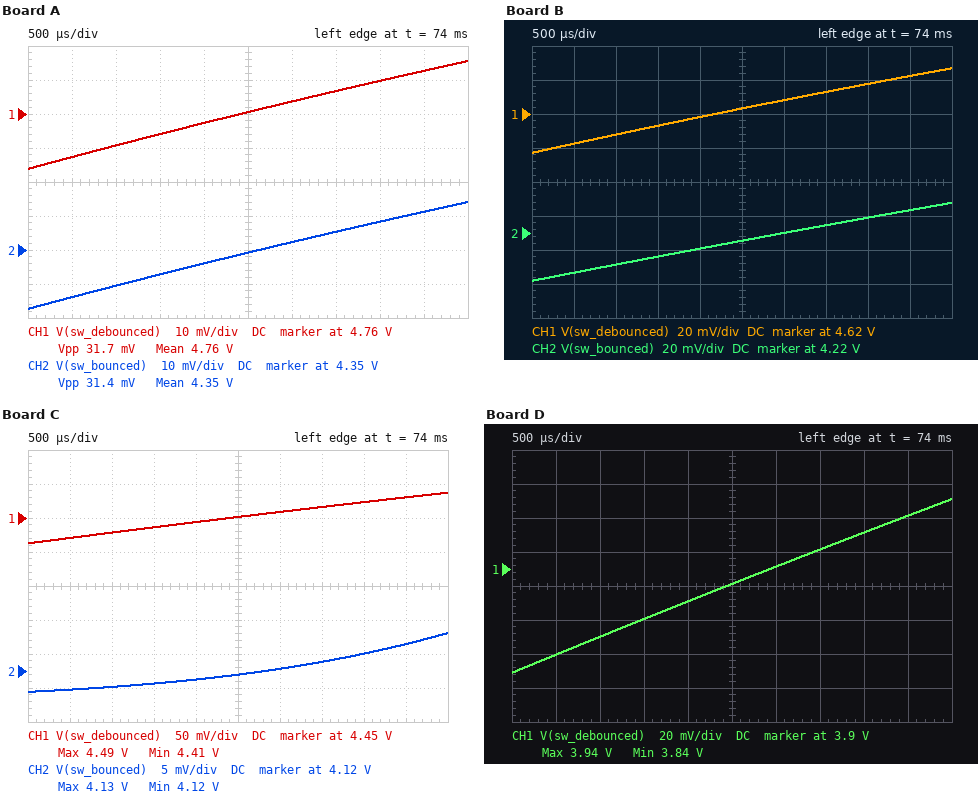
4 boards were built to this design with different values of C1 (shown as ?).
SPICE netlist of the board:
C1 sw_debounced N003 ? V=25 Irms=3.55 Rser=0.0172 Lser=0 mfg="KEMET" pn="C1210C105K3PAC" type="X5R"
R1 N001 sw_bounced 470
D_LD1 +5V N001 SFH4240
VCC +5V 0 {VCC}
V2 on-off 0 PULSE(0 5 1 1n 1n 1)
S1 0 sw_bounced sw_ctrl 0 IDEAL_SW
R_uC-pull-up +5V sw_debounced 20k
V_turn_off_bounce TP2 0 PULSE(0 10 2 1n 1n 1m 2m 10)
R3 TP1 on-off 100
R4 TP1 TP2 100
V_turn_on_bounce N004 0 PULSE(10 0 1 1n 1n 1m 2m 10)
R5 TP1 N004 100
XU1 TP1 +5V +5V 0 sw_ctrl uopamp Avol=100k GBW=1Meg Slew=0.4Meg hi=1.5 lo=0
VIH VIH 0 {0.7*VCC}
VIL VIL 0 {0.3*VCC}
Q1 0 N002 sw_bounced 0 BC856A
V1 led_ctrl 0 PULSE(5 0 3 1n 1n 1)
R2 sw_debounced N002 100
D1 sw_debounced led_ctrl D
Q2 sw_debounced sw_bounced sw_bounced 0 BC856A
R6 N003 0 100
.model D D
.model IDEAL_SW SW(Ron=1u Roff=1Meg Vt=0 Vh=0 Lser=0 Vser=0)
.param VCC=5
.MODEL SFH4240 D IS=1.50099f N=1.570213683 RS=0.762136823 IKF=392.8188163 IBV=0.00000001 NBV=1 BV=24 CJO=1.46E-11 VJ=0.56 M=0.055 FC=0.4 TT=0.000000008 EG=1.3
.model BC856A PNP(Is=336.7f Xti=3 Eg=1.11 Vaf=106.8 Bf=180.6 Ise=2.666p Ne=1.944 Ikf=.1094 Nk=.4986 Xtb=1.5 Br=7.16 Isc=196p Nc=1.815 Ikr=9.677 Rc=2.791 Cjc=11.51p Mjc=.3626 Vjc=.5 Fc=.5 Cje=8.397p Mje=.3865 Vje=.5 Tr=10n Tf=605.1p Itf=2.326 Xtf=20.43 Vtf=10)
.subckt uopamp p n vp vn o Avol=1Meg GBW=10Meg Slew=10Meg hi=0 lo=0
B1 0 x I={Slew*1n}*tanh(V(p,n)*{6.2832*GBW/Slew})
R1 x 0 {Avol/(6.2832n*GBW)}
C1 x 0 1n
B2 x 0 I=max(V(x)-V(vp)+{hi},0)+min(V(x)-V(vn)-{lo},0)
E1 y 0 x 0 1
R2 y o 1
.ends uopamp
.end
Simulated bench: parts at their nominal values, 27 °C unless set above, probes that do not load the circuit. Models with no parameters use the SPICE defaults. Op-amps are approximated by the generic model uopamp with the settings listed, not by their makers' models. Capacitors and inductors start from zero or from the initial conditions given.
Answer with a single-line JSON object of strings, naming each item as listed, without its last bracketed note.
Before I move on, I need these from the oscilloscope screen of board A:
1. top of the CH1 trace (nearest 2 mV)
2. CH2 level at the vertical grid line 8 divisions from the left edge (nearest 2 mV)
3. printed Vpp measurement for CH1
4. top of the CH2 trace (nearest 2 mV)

{"top of the CH1 trace": "4.776 V", "CH2 level at the vertical grid line 8 divisions from the left edge": "4.358 V", "printed Vpp measurement for CH1": "31.7 mV", "top of the CH2 trace": "4.364 V"}
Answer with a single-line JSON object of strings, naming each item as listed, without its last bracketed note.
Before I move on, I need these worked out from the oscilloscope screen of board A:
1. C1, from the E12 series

{"C1, from the E12 series": "1.2 µF"}
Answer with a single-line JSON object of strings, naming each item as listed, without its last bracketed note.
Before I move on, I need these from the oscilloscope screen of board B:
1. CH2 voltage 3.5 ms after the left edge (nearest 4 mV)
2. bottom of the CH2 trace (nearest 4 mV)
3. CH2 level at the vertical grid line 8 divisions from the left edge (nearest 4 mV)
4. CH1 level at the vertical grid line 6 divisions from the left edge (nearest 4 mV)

{"CH2 voltage 3.5 ms after the left edge": "4.224 V", "bottom of the CH2 trace": "4.192 V", "CH2 level at the vertical grid line 8 divisions from the left edge": "4.228 V", "CH1 level at the vertical grid line 6 divisions from the left edge": "4.628 V"}
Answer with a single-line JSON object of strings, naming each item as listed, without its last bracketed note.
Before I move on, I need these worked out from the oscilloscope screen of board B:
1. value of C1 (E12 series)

{"value of C1": "1.5 µF"}
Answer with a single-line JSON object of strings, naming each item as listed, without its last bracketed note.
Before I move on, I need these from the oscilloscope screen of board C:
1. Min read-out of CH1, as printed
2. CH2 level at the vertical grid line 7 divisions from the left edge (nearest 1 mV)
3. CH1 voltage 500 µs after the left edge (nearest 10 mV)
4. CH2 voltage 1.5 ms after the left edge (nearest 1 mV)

{"Min read-out of CH1, as printed": "4.41 V", "CH2 level at the vertical grid line 7 divisions from the left edge": "4.121 V", "CH1 voltage 500 µs after the left edge": "4.42 V", "CH2 voltage 1.5 ms after the left edge": "4.118 V"}
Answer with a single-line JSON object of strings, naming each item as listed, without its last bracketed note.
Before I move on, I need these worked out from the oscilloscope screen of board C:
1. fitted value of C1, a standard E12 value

{"fitted value of C1, a standard E12 value": "1.8 µF"}
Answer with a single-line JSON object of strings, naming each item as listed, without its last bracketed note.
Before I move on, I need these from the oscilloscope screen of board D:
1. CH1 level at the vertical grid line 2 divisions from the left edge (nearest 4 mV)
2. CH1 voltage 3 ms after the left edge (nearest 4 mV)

{"CH1 level at the vertical grid line 2 divisions from the left edge": "3.860 V", "CH1 voltage 3 ms after the left edge": "3.900 V"}
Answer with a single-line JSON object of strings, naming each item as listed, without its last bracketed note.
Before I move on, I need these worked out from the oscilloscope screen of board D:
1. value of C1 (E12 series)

{"value of C1": "2.7 µF"}
